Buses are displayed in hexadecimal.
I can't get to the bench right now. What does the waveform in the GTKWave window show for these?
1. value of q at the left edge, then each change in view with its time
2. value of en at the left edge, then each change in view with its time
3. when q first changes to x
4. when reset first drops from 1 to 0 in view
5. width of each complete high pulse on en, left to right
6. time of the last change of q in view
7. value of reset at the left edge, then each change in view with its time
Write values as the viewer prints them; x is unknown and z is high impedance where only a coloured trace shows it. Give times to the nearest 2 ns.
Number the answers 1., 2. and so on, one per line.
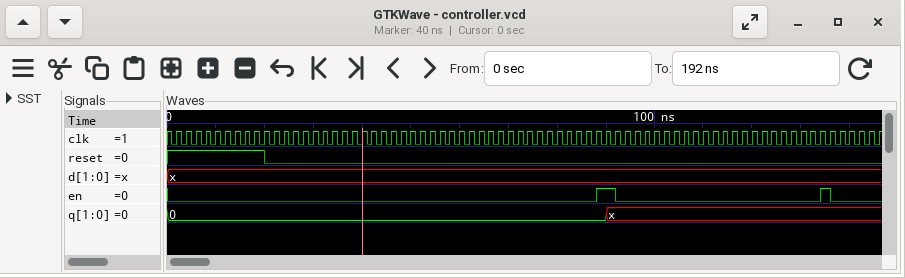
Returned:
1. 0, x at 90 ns
2. 0, 1 at 88 ns, 0 at 92 ns, 1 at 134 ns, 0 at 136 ns
3. 90 ns
4. 20 ns
5. 4 ns, 2 ns
6. 90 ns
7. 1, 0 at 20 ns
